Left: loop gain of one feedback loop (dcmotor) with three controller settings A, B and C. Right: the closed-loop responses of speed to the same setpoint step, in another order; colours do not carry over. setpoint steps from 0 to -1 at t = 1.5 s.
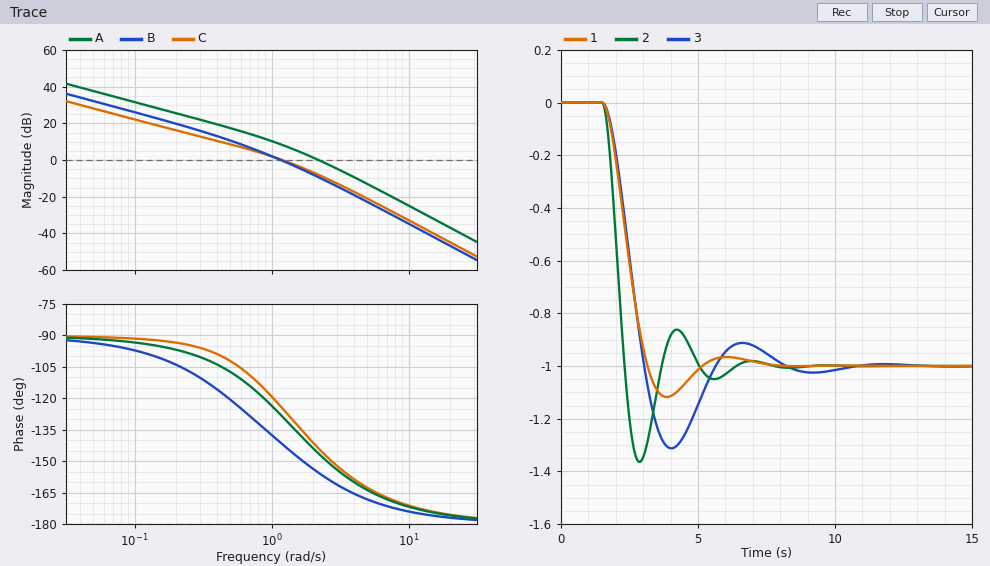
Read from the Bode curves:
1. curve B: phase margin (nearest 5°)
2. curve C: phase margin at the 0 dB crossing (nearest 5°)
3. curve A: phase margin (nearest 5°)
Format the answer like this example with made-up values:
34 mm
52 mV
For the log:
40°
55°
35°
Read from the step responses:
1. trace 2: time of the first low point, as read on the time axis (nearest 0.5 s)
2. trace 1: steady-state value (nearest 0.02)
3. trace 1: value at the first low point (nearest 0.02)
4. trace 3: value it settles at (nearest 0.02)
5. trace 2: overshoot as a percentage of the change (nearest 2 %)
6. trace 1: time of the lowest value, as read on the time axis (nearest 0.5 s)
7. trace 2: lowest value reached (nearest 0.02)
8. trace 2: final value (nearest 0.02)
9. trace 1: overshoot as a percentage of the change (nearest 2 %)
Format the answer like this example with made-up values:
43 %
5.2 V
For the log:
3.0 s
-1.00
-1.12
-1.00
36 %
4.0 s
-1.36
-1.00
12 %
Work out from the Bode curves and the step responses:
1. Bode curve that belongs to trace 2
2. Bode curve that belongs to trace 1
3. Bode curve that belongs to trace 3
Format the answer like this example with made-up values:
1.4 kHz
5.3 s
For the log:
A
C
B
